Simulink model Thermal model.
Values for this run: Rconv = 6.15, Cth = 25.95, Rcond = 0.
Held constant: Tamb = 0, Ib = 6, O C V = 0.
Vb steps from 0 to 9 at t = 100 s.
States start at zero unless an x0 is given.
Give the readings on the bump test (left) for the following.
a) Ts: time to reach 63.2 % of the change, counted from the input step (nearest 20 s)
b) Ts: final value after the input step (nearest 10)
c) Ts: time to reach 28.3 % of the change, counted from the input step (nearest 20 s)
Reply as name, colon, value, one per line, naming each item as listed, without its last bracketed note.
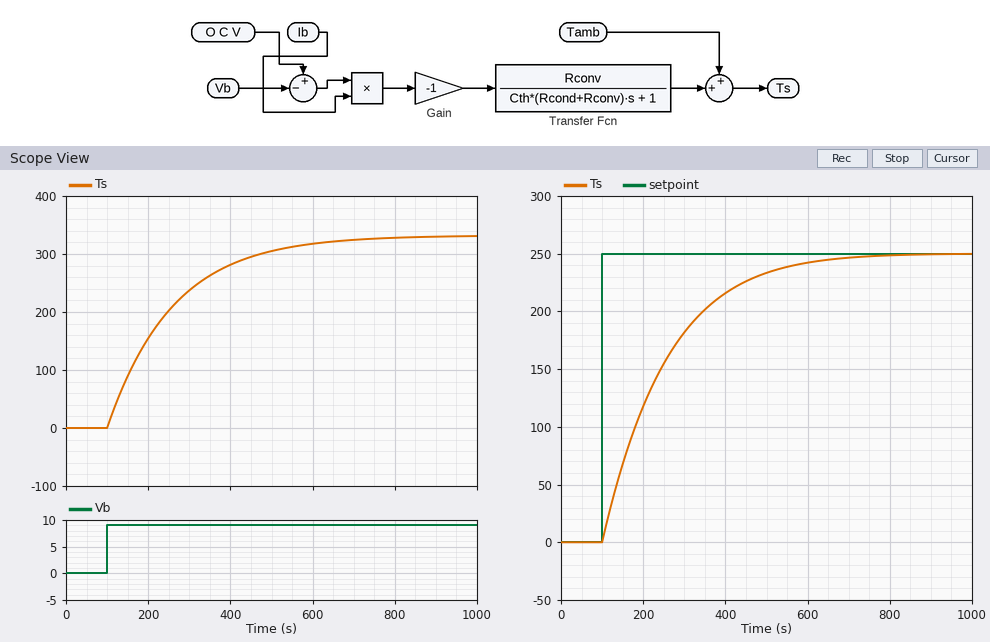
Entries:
Ts: time to reach 63.2 % of the change, counted from the input step: 160 s
Ts: final value after the input step: 330
Ts: time to reach 28.3 % of the change, counted from the input step: 60 s
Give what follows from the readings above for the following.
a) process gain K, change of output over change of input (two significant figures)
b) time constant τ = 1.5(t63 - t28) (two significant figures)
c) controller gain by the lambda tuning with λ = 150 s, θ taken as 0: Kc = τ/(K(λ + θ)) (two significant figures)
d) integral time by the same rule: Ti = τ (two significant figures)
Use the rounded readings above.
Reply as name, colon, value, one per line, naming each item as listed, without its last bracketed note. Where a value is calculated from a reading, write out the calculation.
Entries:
process gain K, change of output over change of input: (330 - 0) / 9 = 37
time constant τ = 1.5(t63 - t28): 1.5 × (160 - 60) = 150 s
controller gain by the lambda tuning with λ = 150 s, θ taken as 0: Kc = τ/(K(λ + θ)): 150 / (37 × (150 + 0)) = 0.027
integral time by the same rule: Ti = τ: 150 s
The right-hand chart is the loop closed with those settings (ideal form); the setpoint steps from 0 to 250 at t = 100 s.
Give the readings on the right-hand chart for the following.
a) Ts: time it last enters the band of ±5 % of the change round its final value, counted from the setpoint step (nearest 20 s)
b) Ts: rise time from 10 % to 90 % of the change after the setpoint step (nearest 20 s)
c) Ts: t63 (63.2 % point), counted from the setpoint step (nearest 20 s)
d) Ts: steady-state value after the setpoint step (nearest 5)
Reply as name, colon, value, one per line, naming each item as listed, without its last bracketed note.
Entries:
Ts: time it last enters the band of ±5 % of the change round its final value, counted from the setpoint step: 440 s
Ts: rise time from 10 % to 90 % of the change after the setpoint step: 320 s
Ts: t63 (63.2 % point), counted from the setpoint step: 160 s
Ts: steady-state value after the setpoint step: 250
